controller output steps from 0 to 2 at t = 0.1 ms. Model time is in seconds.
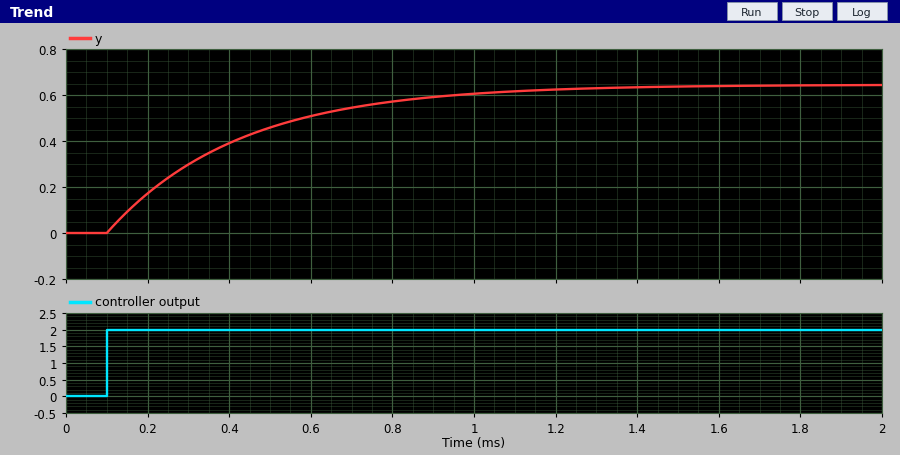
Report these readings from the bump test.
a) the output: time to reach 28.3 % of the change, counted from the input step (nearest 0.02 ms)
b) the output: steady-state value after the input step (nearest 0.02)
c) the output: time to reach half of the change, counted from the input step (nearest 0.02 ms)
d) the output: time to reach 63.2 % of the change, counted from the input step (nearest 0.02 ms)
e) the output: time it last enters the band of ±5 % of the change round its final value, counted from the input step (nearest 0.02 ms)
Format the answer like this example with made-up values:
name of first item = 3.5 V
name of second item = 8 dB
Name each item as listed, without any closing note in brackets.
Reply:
the output: time to reach 28.3 % of the change, counted from the input step = 0.10 ms
the output: steady-state value after the input step = 0.64
the output: time to reach half of the change, counted from the input step = 0.22 ms
the output: time to reach 63.2 % of the change, counted from the input step = 0.32 ms
the output: time it last enters the band of ±5 % of the change round its final value, counted from the input step = 0.96 ms
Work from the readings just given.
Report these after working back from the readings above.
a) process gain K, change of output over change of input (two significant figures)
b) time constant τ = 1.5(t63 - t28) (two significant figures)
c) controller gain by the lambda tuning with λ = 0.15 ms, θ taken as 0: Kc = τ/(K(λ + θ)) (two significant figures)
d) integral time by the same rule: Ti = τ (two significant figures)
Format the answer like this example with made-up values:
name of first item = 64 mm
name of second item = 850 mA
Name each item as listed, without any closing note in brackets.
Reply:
process gain K, change of output over change of input = 0.32
time constant τ = 1.5(t63 - t28) = 0.33 ms
controller gain by the lambda tuning with λ = 0.15 ms, θ taken as 0: Kc = τ/(K(λ + θ)) = 6.9
integral time by the same rule: Ti = τ = 0.33 ms
